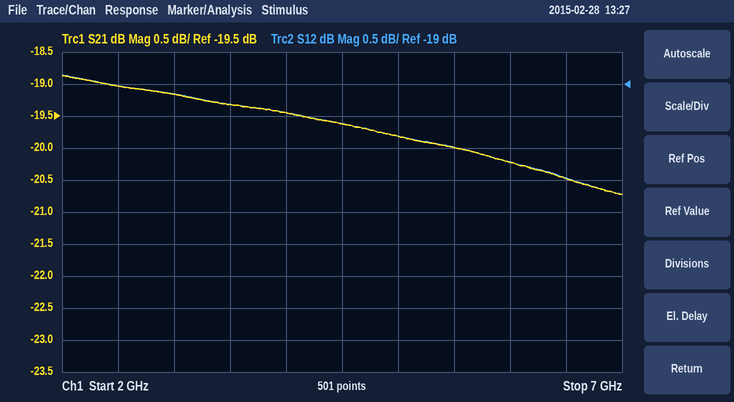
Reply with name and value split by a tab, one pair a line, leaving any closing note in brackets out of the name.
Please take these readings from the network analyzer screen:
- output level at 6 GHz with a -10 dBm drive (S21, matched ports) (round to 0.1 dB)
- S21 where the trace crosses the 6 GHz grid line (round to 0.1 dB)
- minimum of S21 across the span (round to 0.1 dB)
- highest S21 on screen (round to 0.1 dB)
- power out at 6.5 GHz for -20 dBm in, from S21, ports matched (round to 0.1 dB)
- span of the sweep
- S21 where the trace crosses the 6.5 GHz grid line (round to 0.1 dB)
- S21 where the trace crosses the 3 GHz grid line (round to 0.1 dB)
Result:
output level at 6 GHz with a -10 dBm drive (S21, matched ports)	-30.2 dBm
S21 where the trace crosses the 6 GHz grid line	-20.2 dB
minimum of S21 across the span	-20.7 dB
highest S21 on screen	-18.9 dB
power out at 6.5 GHz for -20 dBm in, from S21, ports matched	-40.5 dBm
span of the sweep	5 GHz
S21 where the trace crosses the 6.5 GHz grid line	-20.5 dB
S21 where the trace crosses the 3 GHz grid line	-19.2 dB
